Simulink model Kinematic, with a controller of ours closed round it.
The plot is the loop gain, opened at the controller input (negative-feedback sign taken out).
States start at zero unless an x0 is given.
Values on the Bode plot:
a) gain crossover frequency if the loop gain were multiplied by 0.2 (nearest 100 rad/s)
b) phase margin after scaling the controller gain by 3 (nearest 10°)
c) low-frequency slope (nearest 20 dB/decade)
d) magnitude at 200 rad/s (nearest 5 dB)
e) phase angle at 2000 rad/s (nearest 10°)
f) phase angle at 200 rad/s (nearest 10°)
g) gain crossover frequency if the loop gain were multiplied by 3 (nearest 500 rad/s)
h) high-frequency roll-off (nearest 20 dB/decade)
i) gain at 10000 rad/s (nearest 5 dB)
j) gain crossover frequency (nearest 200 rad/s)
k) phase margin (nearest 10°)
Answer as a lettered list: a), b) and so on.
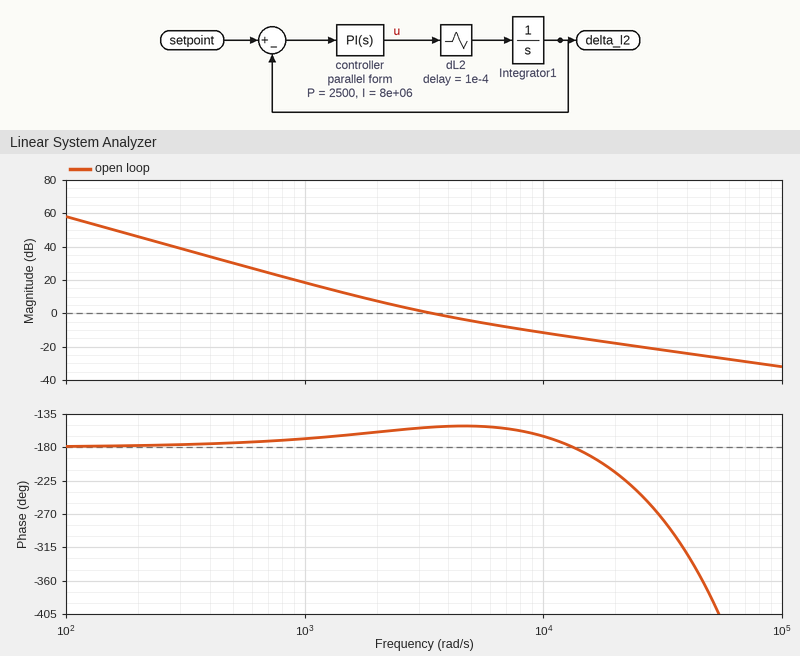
a) 1300 rad/s
b) 20°
c) -40 dB/decade
d) 45 dB
e) -160°
f) -180°
g) 8000 rad/s
h) -20 dB/decade
i) -10 dB
j) 3400 rad/s
k) 30°
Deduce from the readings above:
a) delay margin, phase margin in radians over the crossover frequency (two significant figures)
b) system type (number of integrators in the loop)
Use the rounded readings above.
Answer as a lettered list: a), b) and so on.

a) 0.00015 s
b) 2
